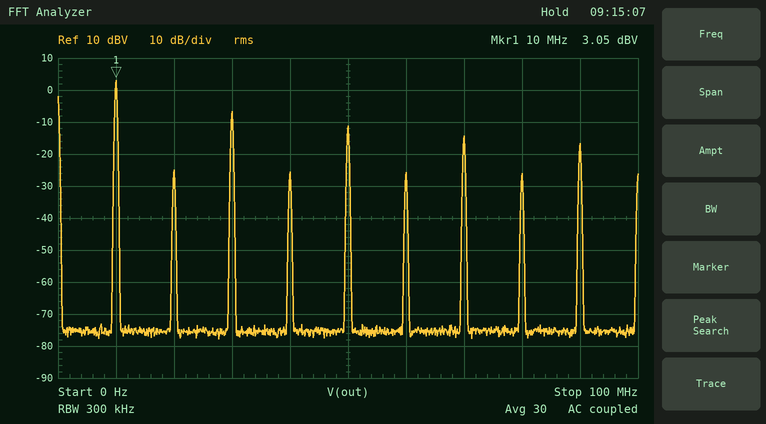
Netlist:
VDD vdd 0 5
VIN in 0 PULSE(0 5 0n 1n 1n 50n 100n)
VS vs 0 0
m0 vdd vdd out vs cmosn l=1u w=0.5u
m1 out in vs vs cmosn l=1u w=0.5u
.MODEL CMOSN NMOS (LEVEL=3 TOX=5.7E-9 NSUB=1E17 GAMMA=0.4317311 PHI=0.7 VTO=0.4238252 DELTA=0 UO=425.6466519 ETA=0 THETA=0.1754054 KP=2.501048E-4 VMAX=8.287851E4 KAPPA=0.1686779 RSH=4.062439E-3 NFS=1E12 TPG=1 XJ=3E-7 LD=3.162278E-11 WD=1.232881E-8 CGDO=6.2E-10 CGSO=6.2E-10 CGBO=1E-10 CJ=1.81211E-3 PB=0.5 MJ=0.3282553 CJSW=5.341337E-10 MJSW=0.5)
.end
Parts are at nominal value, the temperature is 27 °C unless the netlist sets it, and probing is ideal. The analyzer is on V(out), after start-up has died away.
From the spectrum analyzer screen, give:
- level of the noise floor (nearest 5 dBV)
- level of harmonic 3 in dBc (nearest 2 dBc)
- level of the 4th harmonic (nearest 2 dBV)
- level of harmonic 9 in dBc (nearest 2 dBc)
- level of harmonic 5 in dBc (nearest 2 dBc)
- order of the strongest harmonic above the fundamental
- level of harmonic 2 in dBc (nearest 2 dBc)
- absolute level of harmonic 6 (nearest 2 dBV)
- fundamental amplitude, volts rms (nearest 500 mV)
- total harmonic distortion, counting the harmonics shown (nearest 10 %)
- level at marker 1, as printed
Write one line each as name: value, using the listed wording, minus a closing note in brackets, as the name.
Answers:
level of the noise floor: -75 dBV
level of harmonic 3 in dBc: -10 dBc
level of the 4th harmonic: -26 dBV
level of harmonic 9 in dBc: -20 dBc
level of harmonic 5 in dBc: -14 dBc
order of the strongest harmonic above the fundamental: 3
level of harmonic 2 in dBc: -28 dBc
absolute level of harmonic 6: -26 dBV
fundamental amplitude, volts rms: 1.5 V
total harmonic distortion, counting the harmonics shown: 40 %
level at marker 1, as printed: 3.05 dBV
